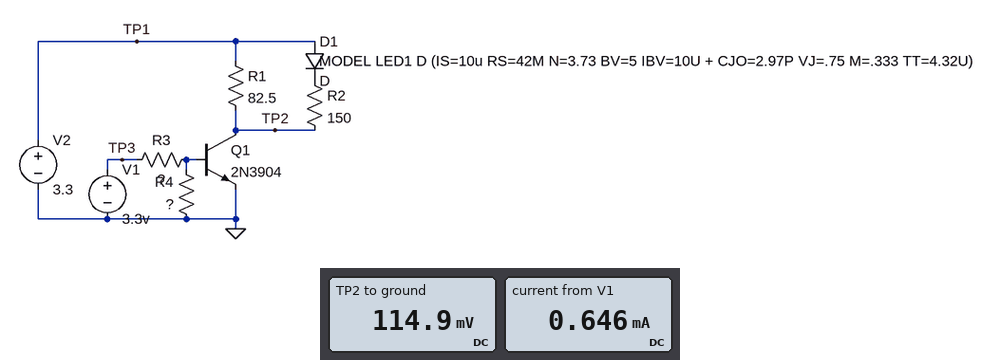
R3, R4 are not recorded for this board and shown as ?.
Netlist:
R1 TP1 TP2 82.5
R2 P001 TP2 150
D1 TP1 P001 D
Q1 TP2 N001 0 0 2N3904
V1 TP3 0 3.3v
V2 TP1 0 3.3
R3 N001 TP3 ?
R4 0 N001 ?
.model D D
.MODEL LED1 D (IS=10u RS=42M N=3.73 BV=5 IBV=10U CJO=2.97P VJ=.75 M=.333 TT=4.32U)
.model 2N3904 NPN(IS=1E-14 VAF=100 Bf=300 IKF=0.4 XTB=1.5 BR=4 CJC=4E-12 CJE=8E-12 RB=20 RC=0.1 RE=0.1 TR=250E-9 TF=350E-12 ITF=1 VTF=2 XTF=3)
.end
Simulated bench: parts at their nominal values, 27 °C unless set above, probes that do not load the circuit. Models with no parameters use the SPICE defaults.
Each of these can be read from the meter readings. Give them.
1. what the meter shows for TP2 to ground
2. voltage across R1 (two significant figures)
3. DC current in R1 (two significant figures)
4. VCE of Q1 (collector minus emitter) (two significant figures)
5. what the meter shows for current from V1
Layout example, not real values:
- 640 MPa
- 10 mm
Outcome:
- 114.9 mV
- 3.2 V
- 39 mA
- 110 mV
- 0.646 mA
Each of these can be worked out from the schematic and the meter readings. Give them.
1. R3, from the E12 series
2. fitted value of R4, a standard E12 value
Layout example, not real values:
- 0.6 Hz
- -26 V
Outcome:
- 3.9 kΩ
- 5.6 kΩ
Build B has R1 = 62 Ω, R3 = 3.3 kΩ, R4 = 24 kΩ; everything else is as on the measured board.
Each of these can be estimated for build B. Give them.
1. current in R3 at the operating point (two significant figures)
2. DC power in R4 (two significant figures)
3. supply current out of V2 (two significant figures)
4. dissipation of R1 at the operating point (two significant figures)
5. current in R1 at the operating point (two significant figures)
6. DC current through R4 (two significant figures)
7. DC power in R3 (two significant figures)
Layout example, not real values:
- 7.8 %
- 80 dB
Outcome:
- 760 µA
- 26 µW
- 68 mA
- 160 mW
- 51 mA
- 33 µA
- 1.9 mW
